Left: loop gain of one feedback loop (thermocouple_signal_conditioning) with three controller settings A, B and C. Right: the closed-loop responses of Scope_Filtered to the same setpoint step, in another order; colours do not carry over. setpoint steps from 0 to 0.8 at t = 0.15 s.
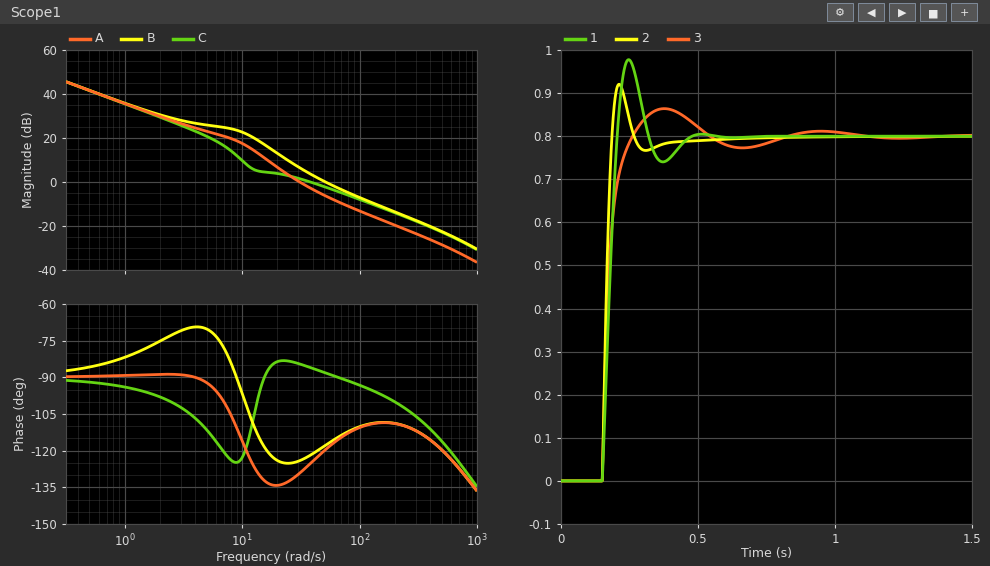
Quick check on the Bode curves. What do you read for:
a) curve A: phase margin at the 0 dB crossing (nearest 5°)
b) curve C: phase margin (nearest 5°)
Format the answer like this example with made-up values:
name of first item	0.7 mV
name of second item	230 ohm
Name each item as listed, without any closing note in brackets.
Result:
curve A: phase margin at the 0 dB crossing	50°
curve C: phase margin	95°
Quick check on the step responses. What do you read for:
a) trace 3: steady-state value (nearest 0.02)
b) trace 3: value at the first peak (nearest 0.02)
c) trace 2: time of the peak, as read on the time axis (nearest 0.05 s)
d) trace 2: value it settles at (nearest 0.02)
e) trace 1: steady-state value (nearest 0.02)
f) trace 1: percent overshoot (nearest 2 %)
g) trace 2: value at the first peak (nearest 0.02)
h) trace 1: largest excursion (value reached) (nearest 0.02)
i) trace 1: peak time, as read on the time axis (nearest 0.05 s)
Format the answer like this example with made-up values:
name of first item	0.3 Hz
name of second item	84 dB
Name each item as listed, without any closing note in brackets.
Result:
trace 3: steady-state value	0.80
trace 3: value at the first peak	0.86
trace 2: time of the peak, as read on the time axis	0.20 s
trace 2: value it settles at	0.80
trace 1: steady-state value	0.80
trace 1: percent overshoot	22 %
trace 2: value at the first peak	0.92
trace 1: largest excursion (value reached)	0.98
trace 1: peak time, as read on the time axis	0.25 s
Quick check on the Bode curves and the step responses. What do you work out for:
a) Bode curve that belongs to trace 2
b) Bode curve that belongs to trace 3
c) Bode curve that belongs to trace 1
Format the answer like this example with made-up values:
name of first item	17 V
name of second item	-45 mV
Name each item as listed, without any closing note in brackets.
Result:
Bode curve that belongs to trace 2	B
Bode curve that belongs to trace 3	C
Bode curve that belongs to trace 1	A
